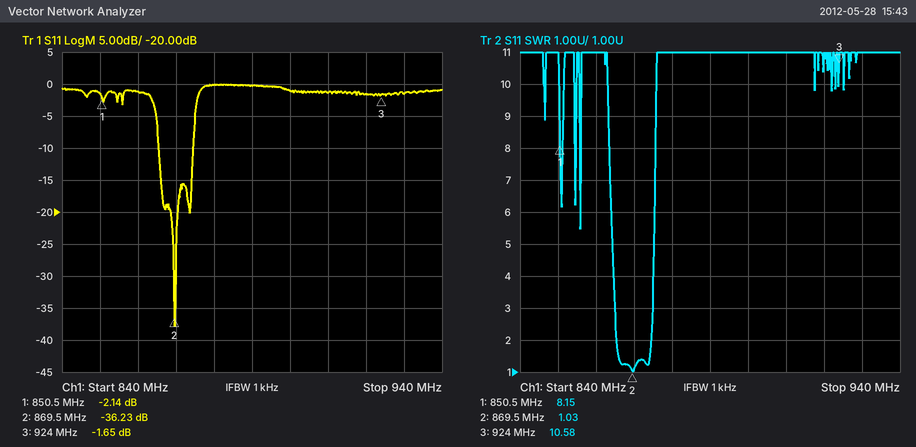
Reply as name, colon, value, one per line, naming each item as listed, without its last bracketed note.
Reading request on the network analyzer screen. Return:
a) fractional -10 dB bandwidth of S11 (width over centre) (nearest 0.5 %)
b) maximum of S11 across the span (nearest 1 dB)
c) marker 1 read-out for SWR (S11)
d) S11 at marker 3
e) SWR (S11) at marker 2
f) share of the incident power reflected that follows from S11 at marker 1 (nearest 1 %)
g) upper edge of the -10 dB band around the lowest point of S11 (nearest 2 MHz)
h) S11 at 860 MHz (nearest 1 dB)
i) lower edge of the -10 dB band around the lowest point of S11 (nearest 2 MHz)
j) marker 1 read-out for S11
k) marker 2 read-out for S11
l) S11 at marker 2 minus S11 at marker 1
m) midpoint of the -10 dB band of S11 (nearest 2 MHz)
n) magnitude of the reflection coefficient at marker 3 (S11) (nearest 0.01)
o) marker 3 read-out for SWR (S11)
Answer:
fractional -10 dB bandwidth of S11 (width over centre): 1.0 %
maximum of S11 across the span: 0 dB
marker 1 read-out for SWR: 8.15
S11 at marker 3: -1.65 dB
SWR (S11) at marker 2: 1.03
share of the incident power reflected that follows from S11 at marker 1: 61 %
upper edge of the -10 dB band around the lowest point of S11: 874 MHz
S11 at 860 MHz: -1 dB
lower edge of the -10 dB band around the lowest point of S11: 866 MHz
marker 1 read-out for S11: -2.14 dB
marker 2 read-out for S11: -36.23 dB
S11 at marker 2 minus S11 at marker 1: -34.09 dB
midpoint of the -10 dB band of S11: 870 MHz
magnitude of the reflection coefficient at marker 3 (S11): 0.83
marker 3 read-out for SWR: 10.58
